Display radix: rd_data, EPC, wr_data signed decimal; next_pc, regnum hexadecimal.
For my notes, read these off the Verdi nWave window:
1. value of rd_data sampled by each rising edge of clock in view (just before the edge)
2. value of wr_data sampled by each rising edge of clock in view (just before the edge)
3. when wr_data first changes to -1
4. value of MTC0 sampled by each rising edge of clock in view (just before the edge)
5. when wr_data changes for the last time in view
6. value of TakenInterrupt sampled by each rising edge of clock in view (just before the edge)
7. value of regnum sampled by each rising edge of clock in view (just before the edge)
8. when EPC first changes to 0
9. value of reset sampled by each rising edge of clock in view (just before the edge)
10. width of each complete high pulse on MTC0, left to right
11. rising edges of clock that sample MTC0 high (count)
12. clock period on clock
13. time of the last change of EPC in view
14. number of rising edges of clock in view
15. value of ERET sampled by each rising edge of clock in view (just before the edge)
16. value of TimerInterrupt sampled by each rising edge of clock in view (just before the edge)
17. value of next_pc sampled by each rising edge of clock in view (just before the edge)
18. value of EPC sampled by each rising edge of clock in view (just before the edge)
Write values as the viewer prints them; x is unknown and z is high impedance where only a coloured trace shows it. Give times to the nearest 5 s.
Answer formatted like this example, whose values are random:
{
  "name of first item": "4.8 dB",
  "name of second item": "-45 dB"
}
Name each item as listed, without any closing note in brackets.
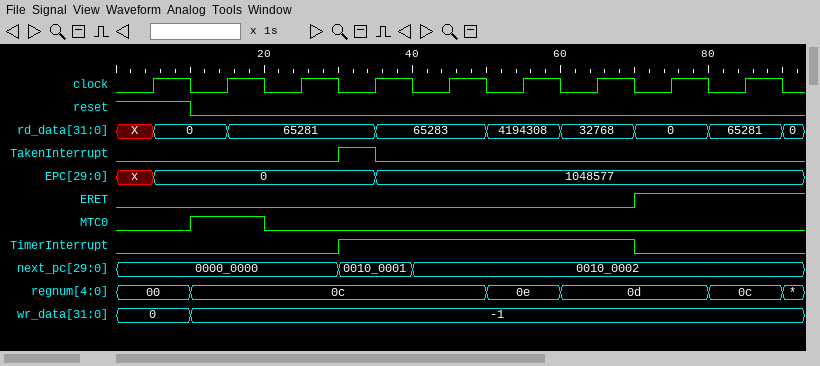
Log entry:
{
  "value of rd_data sampled by each rising edge of clock in view": "X, 0, 65281, 65281, 65283, 4194308, 32768, 0, 65281",
  "value of wr_data sampled by each rising edge of clock in view": "0, -1, -1, -1, -1, -1, -1, -1, -1",
  "when wr_data first changes to -1": "10 s",
  "value of MTC0 sampled by each rising edge of clock in view": "0 1 0 0 0 0 0 0 0",
  "when wr_data changes for the last time in view": "10 s",
  "value of TakenInterrupt sampled by each rising edge of clock in view": "0 0 0 1 0 0 0 0 0",
  "value of regnum sampled by each rising edge of clock in view": "00, 0c, 0c, 0c, 0c, 0e, 0d, 0d, 0c",
  "when EPC first changes to 0": "5 s",
  "value of reset sampled by each rising edge of clock in view": "1 0 0 0 0 0 0 0 0",
  "width of each complete high pulse on MTC0, left to right": "10 s",
  "rising edges of clock that sample MTC0 high": "1",
  "clock period on clock": "10 s",
  "time of the last change of EPC in view": "35 s",
  "number of rising edges of clock in view": "9",
  "value of ERET sampled by each rising edge of clock in view": "0 0 0 0 0 0 0 1 1",
  "value of TimerInterrupt sampled by each rising edge of clock in view": "0 0 0 1 1 1 1 0 0",
  "value of next_pc sampled by each rising edge of clock in view": "0000_0000, 0000_0000, 0000_0000, 0010_0001, 0010_0002, 0010_0002, 0010_0002, 0010_0002, 0010_0002",
  "value of EPC sampled by each rising edge of clock in view": "x, 0, 0, 0, 1048577, 1048577, 1048577, 1048577, 1048577"
}
